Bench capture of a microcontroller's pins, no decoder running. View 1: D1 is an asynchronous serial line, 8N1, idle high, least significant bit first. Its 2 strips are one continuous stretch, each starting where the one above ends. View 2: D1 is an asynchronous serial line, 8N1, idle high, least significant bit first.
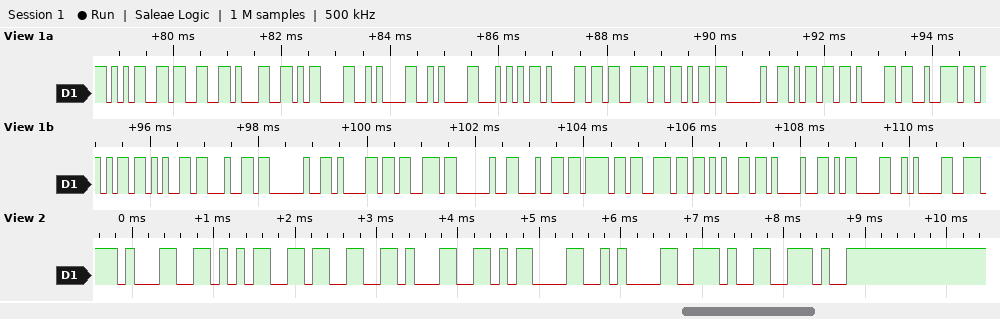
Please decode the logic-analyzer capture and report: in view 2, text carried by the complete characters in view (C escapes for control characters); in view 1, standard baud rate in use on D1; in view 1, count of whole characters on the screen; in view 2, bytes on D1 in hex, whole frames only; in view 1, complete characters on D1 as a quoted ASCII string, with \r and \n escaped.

"1531\r\n.."
9600 baud
28
31 35 33 31 0D 0A 2E 2E
"531\r\n\nTask marked as done!\r\n"
